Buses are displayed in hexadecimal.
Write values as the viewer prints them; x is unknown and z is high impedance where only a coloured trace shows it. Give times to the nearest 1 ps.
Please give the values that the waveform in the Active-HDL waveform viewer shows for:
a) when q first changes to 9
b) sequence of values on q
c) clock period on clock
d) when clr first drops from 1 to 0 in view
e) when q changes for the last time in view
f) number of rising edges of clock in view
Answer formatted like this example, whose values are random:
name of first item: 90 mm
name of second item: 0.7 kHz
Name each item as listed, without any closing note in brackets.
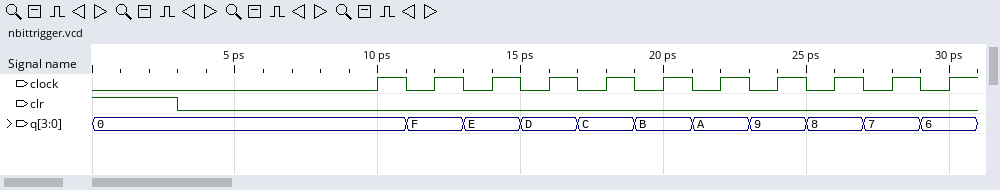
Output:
when q first changes to 9: 23 ps
sequence of values on q: 0, F, E, D, C, B, A, 9, 8, 7, 6
clock period on clock: 2 ps
when clr first drops from 1 to 0 in view: 3 ps
when q changes for the last time in view: 29 ps
number of rising edges of clock in view: 11
